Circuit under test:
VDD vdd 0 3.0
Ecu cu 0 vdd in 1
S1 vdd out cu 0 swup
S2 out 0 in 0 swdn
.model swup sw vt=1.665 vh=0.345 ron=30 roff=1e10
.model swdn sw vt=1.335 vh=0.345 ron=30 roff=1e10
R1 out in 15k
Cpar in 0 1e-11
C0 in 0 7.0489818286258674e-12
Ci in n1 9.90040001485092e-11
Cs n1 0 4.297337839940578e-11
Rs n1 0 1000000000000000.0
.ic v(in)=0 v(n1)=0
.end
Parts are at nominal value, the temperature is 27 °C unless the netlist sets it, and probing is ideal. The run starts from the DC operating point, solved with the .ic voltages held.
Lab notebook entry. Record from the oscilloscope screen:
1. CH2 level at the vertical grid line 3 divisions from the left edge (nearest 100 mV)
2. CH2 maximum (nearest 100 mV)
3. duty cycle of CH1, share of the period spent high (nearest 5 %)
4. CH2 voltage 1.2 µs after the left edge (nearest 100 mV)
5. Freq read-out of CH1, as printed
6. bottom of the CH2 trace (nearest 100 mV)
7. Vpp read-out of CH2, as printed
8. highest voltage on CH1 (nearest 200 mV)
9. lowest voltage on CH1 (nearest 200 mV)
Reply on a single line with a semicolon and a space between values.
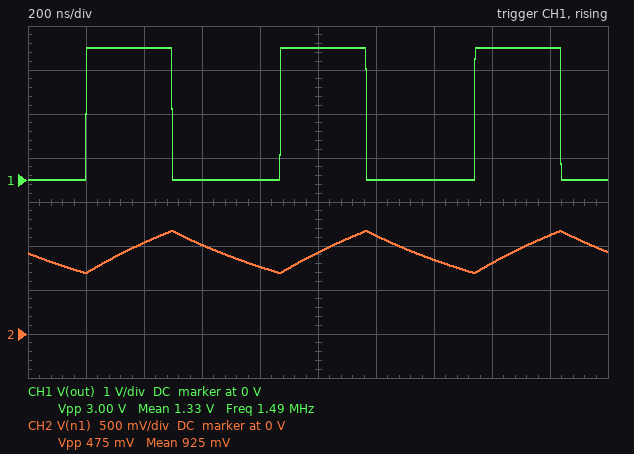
1.0 V; 1.2 V; 45 %; 1.1 V; 1.49 MHz; 700 mV; 475 mV; 3.0 V; 0 V
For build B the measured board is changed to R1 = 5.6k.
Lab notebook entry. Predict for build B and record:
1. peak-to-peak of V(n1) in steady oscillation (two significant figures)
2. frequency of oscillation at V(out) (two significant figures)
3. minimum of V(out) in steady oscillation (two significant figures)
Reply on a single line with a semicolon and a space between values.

480 mV; 4.0 MHz; 5.3 mV
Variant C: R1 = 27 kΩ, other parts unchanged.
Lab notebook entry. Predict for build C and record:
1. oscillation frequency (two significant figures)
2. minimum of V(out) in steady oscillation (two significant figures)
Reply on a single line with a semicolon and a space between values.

830 kHz; 1.1 mV
